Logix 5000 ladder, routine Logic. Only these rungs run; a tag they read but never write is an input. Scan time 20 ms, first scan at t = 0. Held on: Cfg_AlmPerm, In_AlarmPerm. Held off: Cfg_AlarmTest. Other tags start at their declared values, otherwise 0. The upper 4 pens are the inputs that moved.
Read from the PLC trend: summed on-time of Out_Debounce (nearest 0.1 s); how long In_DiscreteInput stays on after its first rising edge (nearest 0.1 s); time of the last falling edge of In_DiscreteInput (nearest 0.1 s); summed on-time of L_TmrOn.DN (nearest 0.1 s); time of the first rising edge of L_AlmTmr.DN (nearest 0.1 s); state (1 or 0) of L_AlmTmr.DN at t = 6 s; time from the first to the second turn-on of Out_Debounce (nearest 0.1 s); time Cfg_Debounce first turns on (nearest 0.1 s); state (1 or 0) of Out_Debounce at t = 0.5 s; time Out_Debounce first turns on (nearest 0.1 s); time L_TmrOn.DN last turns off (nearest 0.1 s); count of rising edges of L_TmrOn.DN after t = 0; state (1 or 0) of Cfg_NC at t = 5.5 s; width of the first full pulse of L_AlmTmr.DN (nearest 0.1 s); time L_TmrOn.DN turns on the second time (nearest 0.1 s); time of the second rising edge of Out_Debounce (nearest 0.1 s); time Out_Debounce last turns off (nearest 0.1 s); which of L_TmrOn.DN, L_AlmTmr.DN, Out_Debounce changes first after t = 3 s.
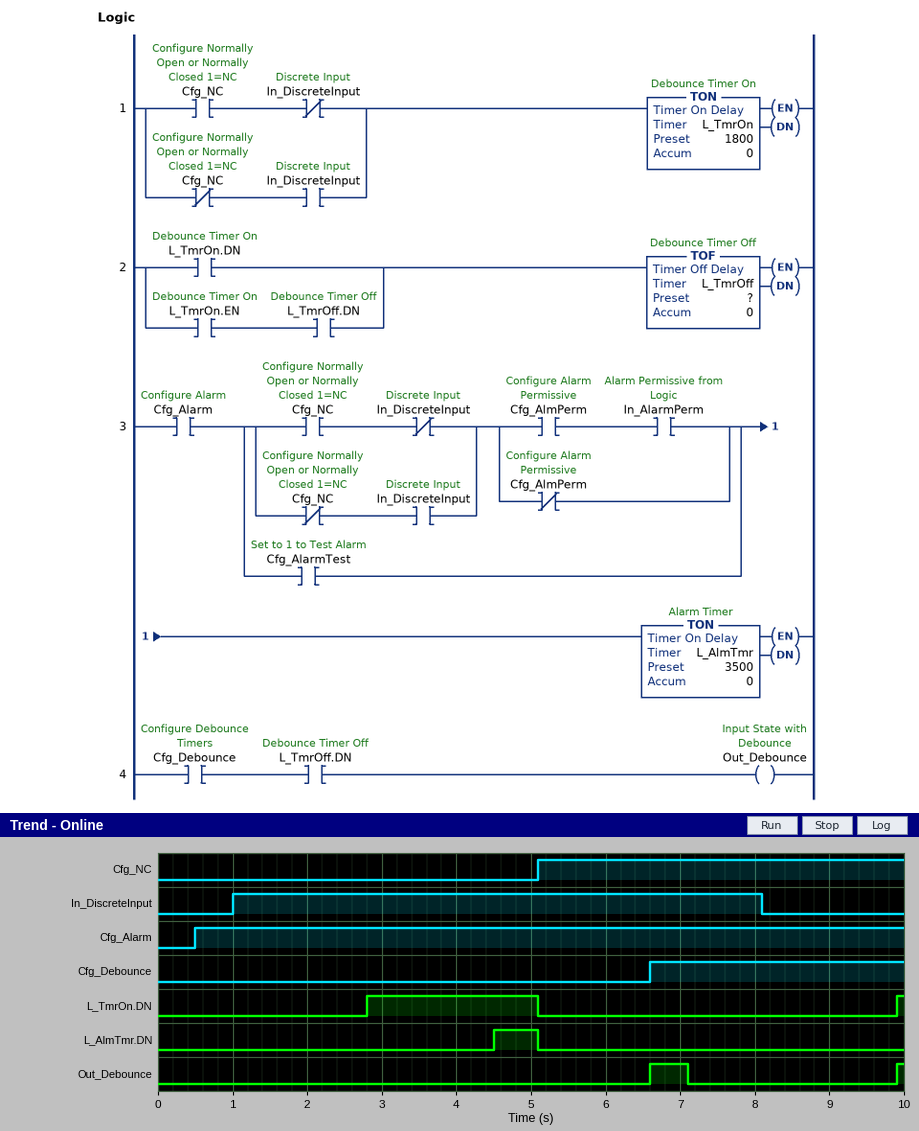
0.6 s
7.1 s
8.1 s
2.4 s
4.5 s
0
3.3 s
6.6 s
0
6.6 s
5.1 s
2
1
0.6 s
9.9 s
9.9 s
7.1 s
L_AlmTmr.DN
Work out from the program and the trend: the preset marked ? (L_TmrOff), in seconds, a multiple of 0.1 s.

2.0 s
